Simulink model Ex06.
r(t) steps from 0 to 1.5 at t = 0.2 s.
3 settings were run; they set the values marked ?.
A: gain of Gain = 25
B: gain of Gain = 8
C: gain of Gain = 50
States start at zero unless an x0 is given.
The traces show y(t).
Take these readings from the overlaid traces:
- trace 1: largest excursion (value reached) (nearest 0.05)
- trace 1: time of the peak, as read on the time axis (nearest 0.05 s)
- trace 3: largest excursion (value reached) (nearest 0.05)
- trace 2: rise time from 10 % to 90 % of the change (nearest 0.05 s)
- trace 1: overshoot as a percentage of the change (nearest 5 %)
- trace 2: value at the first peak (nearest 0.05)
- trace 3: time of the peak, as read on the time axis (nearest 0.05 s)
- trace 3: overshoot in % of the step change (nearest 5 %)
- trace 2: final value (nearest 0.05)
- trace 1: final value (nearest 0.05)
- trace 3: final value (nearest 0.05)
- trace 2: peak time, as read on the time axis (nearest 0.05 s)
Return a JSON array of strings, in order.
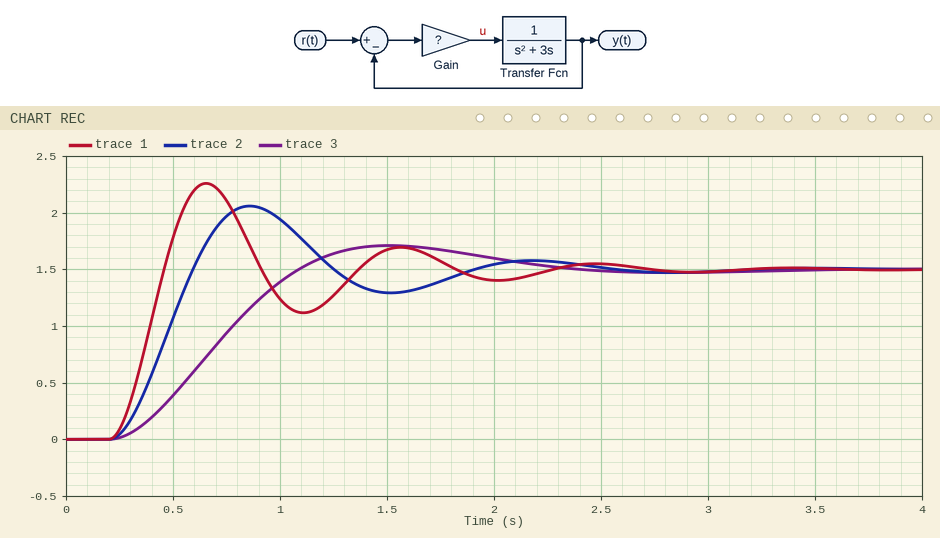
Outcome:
["2.25", "0.65 s", "1.70", "0.25 s", "50 %", "2.05", "1.50 s", "15 %", "1.50", "1.50", "1.50", "0.85 s"]
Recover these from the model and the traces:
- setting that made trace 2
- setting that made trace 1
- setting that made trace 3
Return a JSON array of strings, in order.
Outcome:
["A", "C", "B"]
